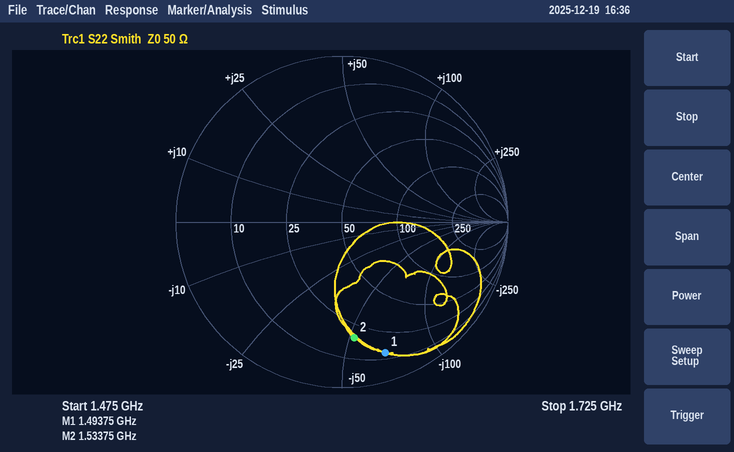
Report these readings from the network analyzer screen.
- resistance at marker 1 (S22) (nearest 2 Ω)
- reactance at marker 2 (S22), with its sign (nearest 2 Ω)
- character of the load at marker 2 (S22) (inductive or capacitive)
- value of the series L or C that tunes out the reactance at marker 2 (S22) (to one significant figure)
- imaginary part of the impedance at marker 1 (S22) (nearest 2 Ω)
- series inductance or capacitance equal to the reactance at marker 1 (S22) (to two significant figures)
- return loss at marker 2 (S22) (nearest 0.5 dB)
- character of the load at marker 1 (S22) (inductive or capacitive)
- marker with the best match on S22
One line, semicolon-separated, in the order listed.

14 Ω; -52 Ω; capacitive; 5 nH; -68 Ω; 1.6 pF; 3.0 dB; capacitive; marker 2
